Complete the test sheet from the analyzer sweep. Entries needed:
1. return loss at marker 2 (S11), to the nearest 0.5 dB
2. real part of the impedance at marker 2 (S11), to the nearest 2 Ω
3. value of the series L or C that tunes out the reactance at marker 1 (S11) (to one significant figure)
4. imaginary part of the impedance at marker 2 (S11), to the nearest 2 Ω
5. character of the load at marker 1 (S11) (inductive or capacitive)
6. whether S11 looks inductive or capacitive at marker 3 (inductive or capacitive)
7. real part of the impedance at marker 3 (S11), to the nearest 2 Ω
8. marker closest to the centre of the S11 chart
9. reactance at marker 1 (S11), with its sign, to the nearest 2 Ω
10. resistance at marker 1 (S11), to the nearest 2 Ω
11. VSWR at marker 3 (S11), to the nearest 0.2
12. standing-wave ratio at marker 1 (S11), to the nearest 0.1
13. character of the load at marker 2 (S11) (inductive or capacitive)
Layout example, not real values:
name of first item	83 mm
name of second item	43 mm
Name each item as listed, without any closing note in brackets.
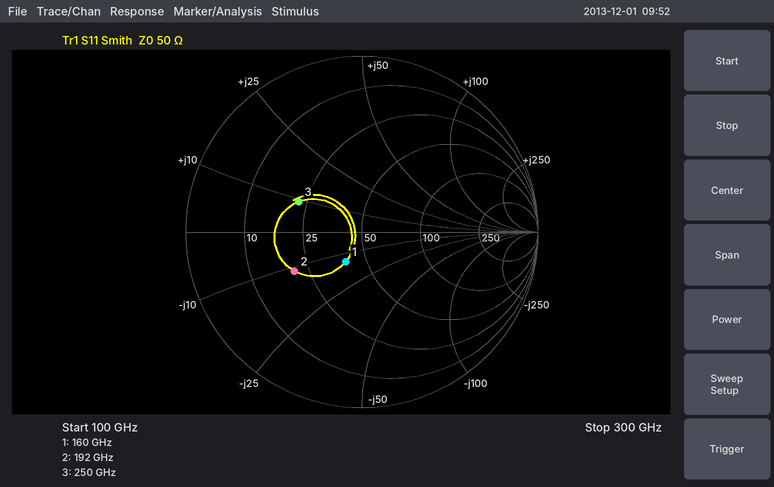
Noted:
return loss at marker 2 (S11), to the nearest 0.5 dB	7.0 dB
real part of the impedance at marker 2 (S11), to the nearest 2 Ω	20 Ω
value of the series L or C that tunes out the reactance at marker 1 (S11)	10 pH
imaginary part of the impedance at marker 2 (S11), to the nearest 2 Ω	-12 Ω
character of the load at marker 1 (S11)	capacitive
whether S11 looks inductive or capacitive at marker 3	inductive
real part of the impedance at marker 3 (S11), to the nearest 2 Ω	22 Ω
marker closest to the centre of the S11 chart	marker 1
reactance at marker 1 (S11), with its sign, to the nearest 2 Ω	-14 Ω
resistance at marker 1 (S11), to the nearest 2 Ω	40 Ω
VSWR at marker 3 (S11), to the nearest 0.2	2.4
standing-wave ratio at marker 1 (S11), to the nearest 0.1	1.5
character of the load at marker 2 (S11)	capacitive
